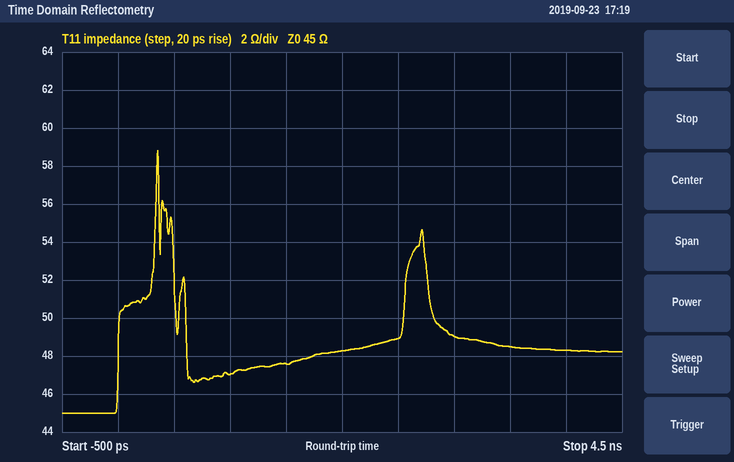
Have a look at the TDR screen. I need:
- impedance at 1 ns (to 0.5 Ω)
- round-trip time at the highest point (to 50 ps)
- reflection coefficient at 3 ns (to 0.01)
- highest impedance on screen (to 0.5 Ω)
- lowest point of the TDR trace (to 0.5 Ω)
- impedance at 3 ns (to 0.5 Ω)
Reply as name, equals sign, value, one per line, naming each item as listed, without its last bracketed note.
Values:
impedance at 1 ns = 47.0 Ω
round-trip time at the highest point = 350 ps
reflection coefficient at 3 ns = +0.04
highest impedance on screen = 59.0 Ω
lowest point of the TDR trace = 45.0 Ω
impedance at 3 ns = 49.0 Ω
